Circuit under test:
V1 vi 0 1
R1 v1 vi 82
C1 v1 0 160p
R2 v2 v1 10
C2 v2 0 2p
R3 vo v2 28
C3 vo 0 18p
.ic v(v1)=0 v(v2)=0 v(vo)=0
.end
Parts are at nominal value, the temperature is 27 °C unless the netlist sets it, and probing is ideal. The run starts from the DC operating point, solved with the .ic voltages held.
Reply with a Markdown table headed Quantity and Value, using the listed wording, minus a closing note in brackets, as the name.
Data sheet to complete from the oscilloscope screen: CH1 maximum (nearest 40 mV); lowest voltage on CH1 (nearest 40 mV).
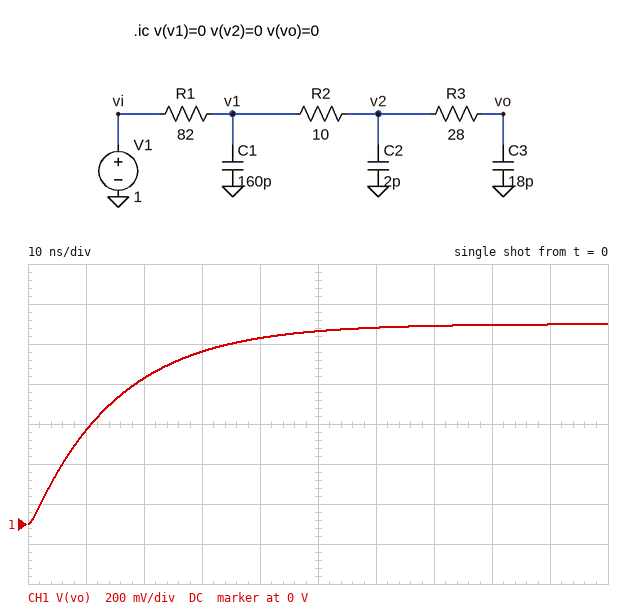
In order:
| Quantity | Value |
|---|---|
| CH1 maximum | 1.00 V |
| lowest voltage on CH1 | 0 V |
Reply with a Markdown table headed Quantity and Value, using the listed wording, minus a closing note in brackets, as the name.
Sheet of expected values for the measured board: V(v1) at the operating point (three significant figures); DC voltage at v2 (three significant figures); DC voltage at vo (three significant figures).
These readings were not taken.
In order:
| Quantity | Value |
|---|---|
| V(v1) at the operating point | 1.00 V |
| DC voltage at v2 | 1.00 V |
| DC voltage at vo | 1.00 V |
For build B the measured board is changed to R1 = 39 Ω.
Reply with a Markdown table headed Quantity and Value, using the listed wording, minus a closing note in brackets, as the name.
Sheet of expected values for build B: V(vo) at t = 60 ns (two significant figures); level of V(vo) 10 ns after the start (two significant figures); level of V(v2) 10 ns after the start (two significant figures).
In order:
| Quantity | Value |
|---|---|
| V(vo) at t = 60 ns | 1.0 V |
| level of V(vo) 10 ns after the start | 730 mV |
| level of V(v2) 10 ns after the start | 750 mV |
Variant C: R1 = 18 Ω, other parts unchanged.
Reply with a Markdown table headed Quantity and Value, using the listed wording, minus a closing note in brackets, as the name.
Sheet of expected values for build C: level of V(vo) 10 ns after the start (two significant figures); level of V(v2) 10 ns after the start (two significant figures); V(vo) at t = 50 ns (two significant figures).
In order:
| Quantity | Value |
|---|---|
| level of V(vo) 10 ns after the start | 940 mV |
| level of V(v2) 10 ns after the start | 950 mV |
| V(vo) at t = 50 ns | 1.0 V |
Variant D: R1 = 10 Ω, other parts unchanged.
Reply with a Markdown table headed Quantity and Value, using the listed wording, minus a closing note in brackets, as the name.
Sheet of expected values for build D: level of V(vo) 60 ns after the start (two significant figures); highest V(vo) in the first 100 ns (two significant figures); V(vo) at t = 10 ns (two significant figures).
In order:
| Quantity | Value |
|---|---|
| level of V(vo) 60 ns after the start | 1.0 V |
| highest V(vo) in the first 100 ns | 1.0 V |
| V(vo) at t = 10 ns | 990 mV |
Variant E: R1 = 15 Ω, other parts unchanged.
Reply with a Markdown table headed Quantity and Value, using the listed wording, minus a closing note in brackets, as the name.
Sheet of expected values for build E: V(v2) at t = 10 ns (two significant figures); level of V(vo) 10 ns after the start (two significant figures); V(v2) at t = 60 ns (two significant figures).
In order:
| Quantity | Value |
|---|---|
| V(v2) at t = 10 ns | 970 mV |
| level of V(vo) 10 ns after the start | 960 mV |
| V(v2) at t = 60 ns | 1.0 V |
